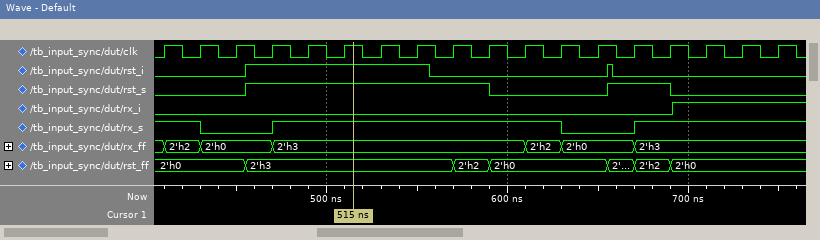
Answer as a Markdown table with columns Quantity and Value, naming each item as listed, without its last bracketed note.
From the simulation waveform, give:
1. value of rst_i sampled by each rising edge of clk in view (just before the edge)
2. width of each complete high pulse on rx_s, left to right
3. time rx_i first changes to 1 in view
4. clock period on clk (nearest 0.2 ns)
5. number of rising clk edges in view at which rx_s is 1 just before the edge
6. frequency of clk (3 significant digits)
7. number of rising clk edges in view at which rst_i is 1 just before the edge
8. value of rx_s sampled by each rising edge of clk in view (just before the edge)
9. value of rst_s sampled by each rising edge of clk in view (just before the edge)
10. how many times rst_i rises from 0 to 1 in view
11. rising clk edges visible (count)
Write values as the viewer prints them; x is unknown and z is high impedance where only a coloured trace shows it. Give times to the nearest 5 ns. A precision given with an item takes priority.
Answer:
| Quantity | Value |
|---|---|
| value of rst_i sampled by each rising edge of clk in view | 0 0 0 1 1 1 1 1 0 0 0 0 0 0 0 0 0 0 |
| width of each complete high pulse on rx_s, left to right | 160 ns |
| time rx_i first changes to 1 in view | 690 ns |
| clock period on clk | 20 ns |
| number of rising clk edges in view at which rx_s is 1 just before the edge | 14 |
| frequency of clk | 50.0 MHz |
| number of rising clk edges in view at which rst_i is 1 just before the edge | 5 |
| value of rx_s sampled by each rising edge of clk in view | 1 1 0 0 1 1 1 1 1 1 1 1 0 0 1 1 1 1 |
| value of rst_s sampled by each rising edge of clk in view | 0 0 0 1 1 1 1 1 1 1 0 0 0 1 1 0 0 0 |
| how many times rst_i rises from 0 to 1 in view | 2 |
| rising clk edges visible | 18 |
